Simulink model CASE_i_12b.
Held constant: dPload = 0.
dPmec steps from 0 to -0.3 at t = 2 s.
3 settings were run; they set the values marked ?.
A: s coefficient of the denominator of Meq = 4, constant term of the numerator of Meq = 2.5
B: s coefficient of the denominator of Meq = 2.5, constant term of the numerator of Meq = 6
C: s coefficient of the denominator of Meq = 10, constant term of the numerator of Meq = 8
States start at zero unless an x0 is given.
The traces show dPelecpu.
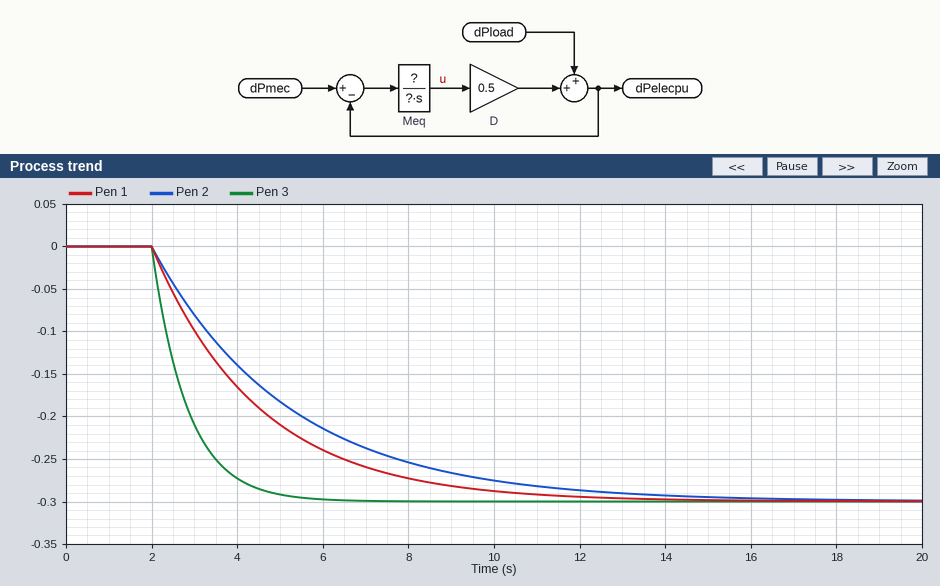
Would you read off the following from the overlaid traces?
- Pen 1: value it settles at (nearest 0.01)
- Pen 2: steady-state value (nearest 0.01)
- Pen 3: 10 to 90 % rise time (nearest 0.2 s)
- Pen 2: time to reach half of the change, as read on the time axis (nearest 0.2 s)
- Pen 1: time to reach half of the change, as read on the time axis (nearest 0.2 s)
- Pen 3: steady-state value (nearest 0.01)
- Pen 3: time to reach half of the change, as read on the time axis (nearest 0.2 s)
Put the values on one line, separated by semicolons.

-0.30; -0.30; 1.8 s; 4.2 s; 3.8 s; -0.30; 2.6 s
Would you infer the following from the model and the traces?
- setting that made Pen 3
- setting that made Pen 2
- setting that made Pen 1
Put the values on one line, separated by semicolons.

B; A; C
